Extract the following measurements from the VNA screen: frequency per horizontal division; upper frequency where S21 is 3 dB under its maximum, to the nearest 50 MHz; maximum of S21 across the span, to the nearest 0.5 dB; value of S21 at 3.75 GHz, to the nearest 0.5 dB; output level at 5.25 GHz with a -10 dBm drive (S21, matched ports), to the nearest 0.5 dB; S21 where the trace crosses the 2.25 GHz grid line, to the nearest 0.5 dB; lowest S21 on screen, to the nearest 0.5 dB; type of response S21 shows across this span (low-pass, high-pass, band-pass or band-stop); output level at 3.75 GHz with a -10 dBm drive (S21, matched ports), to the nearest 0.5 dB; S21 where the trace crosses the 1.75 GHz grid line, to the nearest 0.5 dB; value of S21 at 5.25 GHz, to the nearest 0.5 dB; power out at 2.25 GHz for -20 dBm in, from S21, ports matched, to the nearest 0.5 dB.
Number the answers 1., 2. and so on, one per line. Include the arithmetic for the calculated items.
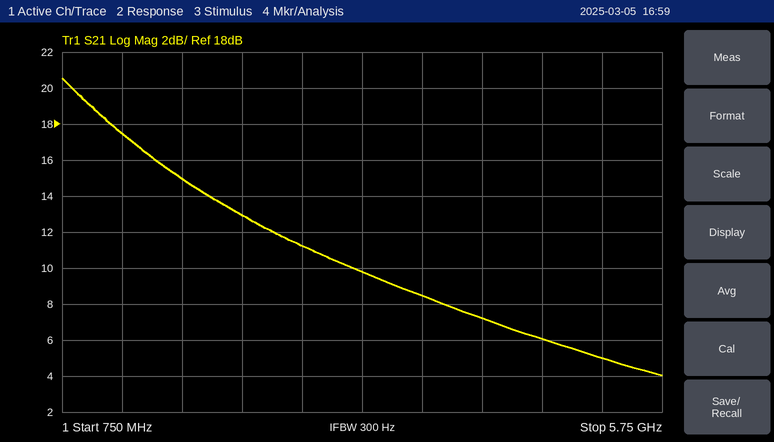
1. 500 MHz
2. 1.25 GHz
3. 20.5 dB
4. 8.5 dB
5. -10 dBm + (5.0 dB) = -5.0 dBm
6. 13.0 dB
7. 4.0 dB
8. low-pass
9. -10 dBm + (8.5 dB) = -1.5 dBm
10. 15.0 dB
11. 5.0 dB
12. -20 dBm + (13.0 dB) = -7.0 dBm
